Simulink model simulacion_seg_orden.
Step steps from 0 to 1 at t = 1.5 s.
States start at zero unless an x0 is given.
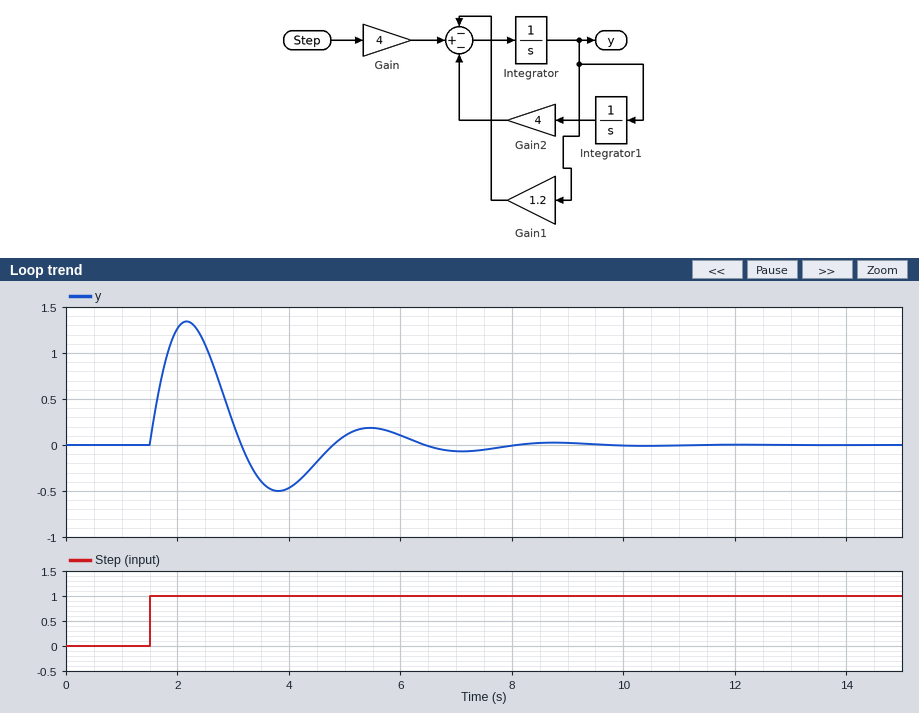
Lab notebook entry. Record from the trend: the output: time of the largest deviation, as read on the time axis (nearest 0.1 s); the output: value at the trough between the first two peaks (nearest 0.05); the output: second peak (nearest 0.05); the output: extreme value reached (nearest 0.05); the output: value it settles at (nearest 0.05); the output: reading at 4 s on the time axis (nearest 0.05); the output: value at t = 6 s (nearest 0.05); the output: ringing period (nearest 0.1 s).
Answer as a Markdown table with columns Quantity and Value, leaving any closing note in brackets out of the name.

| Quantity | Value |
|---|---|
| the output: time of the largest deviation, as read on the time axis | 2.2 s |
| the output: value at the trough between the first two peaks | -0.50 |
| the output: second peak | 0.20 |
| the output: extreme value reached | 1.35 |
| the output: value it settles at | 0.00 |
| the output: reading at 4 s on the time axis | -0.45 |
| the output: value at t = 6 s | 0.10 |
| the output: ringing period | 3.3 s |
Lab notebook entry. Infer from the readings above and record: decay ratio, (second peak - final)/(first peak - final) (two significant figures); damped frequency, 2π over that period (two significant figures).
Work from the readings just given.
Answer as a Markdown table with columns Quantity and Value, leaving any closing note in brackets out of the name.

| Quantity | Value |
|---|---|
| decay ratio, (second peak - final)/(first peak - final) | 0.15 |
| damped frequency, 2π over that period | 1.9 rad/s |
